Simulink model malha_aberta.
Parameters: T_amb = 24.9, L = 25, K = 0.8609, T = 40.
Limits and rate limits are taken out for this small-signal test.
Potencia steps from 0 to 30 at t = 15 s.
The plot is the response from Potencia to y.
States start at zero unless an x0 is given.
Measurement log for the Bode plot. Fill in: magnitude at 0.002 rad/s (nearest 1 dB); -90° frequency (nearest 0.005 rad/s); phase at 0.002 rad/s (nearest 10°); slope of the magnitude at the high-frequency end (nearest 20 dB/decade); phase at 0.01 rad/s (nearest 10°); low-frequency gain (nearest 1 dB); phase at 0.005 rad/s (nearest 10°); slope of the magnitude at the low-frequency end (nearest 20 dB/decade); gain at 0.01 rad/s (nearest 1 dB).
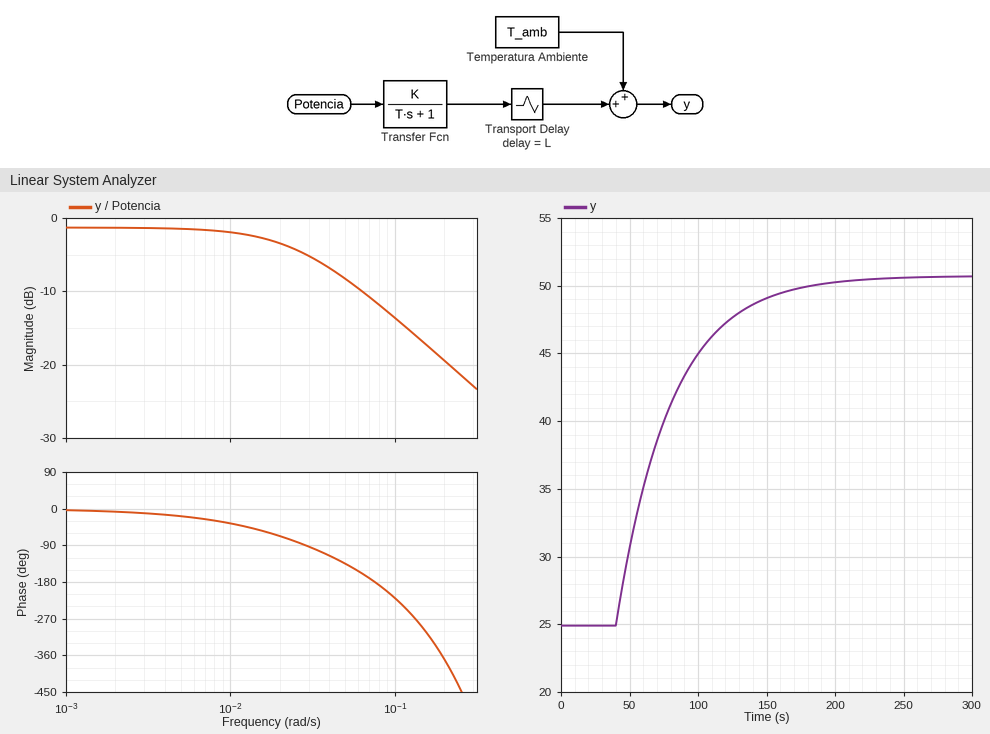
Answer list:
-1 dB
0.030 rad/s
-10°
-20 dB/decade
-40°
-1 dB
-20°
0 dB/decade
-2 dB
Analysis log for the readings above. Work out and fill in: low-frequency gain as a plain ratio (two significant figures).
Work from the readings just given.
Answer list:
0.89
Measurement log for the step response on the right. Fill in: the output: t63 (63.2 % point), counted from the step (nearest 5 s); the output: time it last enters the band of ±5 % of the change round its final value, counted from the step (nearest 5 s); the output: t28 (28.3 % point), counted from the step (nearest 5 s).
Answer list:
65 s
145 s
40 s
